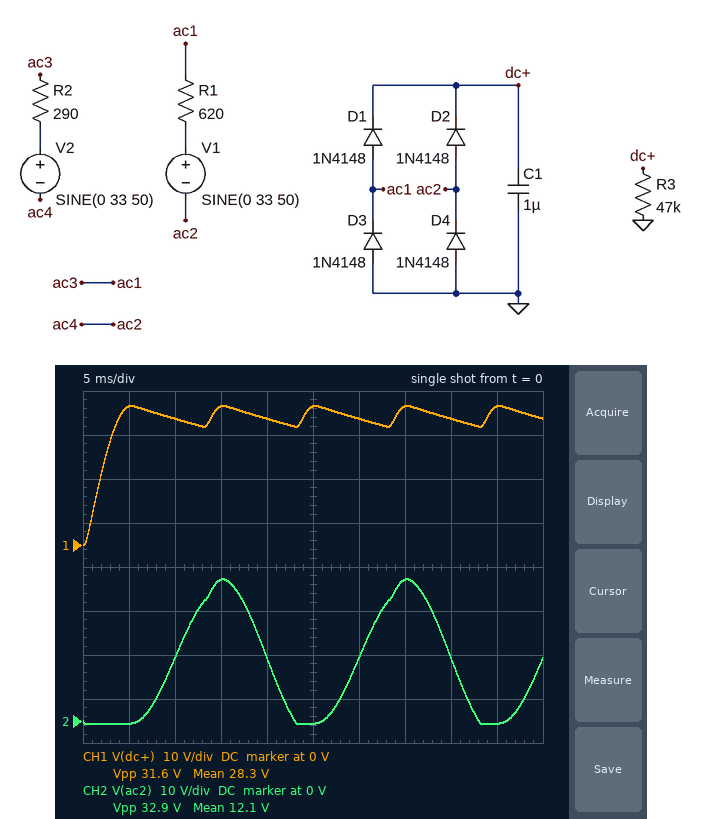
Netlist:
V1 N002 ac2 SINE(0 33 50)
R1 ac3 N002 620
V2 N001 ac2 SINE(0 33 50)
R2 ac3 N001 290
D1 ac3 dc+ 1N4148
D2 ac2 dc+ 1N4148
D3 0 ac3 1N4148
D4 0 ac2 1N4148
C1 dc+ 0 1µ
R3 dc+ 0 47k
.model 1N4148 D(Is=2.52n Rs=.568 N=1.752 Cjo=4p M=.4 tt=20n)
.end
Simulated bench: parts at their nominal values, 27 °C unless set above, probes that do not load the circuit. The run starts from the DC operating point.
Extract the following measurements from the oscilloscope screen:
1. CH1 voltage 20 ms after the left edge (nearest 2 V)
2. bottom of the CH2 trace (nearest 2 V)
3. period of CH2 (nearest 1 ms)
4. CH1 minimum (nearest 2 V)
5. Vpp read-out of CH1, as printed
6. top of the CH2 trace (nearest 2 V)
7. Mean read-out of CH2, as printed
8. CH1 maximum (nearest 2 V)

28 V
0 V
20 ms
0 V
31.6 V
32 V
12.1 V
32 V
